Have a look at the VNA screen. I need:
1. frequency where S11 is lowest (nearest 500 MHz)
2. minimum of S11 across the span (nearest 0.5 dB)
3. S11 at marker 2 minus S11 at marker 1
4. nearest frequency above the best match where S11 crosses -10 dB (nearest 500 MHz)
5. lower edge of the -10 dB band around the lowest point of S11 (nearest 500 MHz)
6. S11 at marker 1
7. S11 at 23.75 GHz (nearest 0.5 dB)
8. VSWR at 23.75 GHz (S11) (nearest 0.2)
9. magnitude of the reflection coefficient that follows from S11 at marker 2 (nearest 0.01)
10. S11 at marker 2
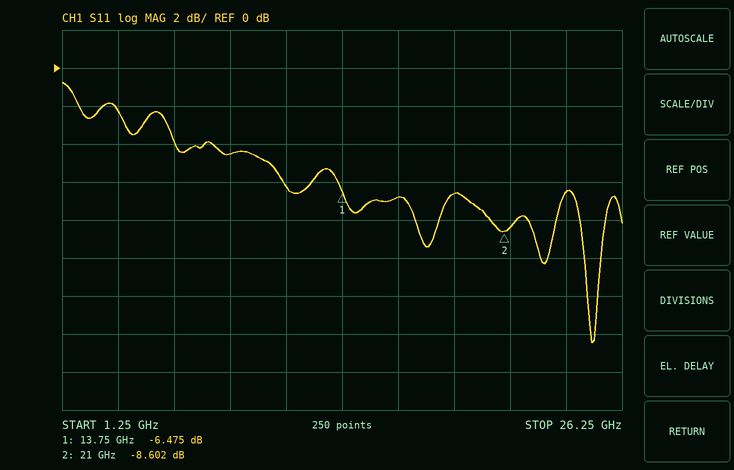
25.0 GHz
-14.5 dB
-2.127 dB
25.5 GHz
24.5 GHz
-6.475 dB
-6.5 dB
2.8
0.37
-8.602 dB
